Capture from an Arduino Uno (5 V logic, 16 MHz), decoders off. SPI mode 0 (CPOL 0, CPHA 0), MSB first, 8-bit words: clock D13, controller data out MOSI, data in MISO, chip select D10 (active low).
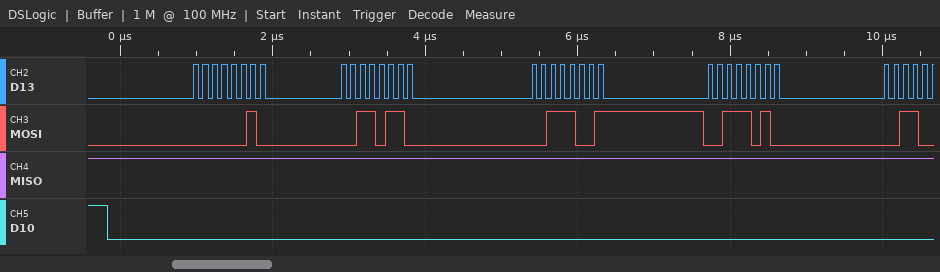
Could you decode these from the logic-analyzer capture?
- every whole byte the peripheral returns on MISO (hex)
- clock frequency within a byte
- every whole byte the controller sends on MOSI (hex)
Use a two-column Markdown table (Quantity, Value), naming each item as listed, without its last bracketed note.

| Quantity | Value |
|---|---|
| every whole byte the peripheral returns on MISO | FF FF FF FF |
| clock frequency within a byte | 8 MHz |
| every whole byte the controller sends on MOSI | 02 36 39 3A |
